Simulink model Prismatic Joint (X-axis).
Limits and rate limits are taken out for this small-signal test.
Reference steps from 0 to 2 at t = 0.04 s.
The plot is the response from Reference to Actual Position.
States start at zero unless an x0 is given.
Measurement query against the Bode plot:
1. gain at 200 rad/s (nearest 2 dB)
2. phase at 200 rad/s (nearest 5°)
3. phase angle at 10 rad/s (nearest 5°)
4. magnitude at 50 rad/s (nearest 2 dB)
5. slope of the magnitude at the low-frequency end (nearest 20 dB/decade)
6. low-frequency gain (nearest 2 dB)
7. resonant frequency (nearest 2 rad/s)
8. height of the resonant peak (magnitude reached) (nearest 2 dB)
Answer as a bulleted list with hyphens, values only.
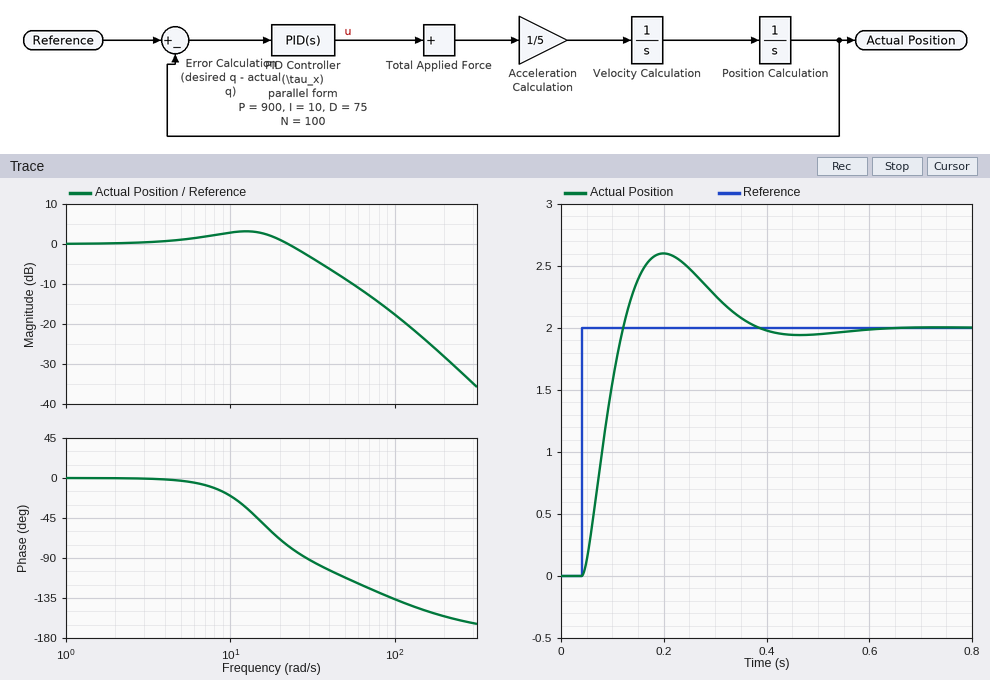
- -28 dB
- -155°
- -20°
- -8 dB
- 0 dB/decade
- 0 dB
- 12 rad/s
- 4 dB
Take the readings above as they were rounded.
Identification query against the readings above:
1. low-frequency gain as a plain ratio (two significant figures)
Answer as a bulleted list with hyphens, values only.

- 1.0
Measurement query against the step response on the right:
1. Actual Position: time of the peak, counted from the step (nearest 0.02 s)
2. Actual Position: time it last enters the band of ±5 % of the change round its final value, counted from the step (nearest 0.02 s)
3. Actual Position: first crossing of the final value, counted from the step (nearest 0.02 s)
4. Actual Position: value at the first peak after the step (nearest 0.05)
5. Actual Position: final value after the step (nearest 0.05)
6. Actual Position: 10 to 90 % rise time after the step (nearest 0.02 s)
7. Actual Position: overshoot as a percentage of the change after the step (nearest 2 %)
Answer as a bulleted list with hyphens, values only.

- 0.16 s
- 0.30 s
- 0.08 s
- 2.60
- 2.00
- 0.06 s
- 30 %
